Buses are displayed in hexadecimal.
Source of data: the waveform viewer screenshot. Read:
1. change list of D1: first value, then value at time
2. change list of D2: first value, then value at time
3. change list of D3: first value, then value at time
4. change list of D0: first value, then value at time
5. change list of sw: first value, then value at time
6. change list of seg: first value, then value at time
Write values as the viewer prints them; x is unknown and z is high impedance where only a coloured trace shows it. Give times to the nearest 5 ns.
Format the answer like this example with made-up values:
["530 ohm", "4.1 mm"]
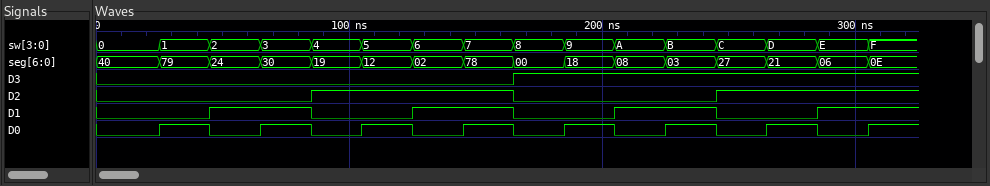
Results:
["0, 1 at 45 ns, 0 at 85 ns, 1 at 125 ns, 0 at 165 ns, 1 at 205 ns, 0 at 245 ns, 1 at 285 ns", "0, 1 at 85 ns, 0 at 165 ns, 1 at 245 ns", "0, 1 at 165 ns", "0, 1 at 25 ns, 0 at 45 ns, 1 at 65 ns, 0 at 85 ns, 1 at 105 ns, 0 at 125 ns, 1 at 145 ns, 0 at 165 ns, 1 at 185 ns, 0 at 205 ns, 1 at 225 ns, 0 at 245 ns, 1 at 265 ns, 0 at 285 ns, 1 at 305 ns", "0, 1 at 25 ns, 2 at 45 ns, 3 at 65 ns, 4 at 85 ns, 5 at 105 ns, 6 at 125 ns, 7 at 145 ns, 8 at 165 ns, 9 at 185 ns, A at 205 ns, B at 225 ns, C at 245 ns, D at 265 ns, E at 285 ns, F at 305 ns", "40, 79 at 25 ns, 24 at 45 ns, 30 at 65 ns, 19 at 85 ns, 12 at 105 ns, 02 at 125 ns, 78 at 145 ns, 00 at 165 ns, 18 at 185 ns, 08 at 205 ns, 03 at 225 ns, 27 at 245 ns, 21 at 265 ns, 06 at 285 ns, 0E at 305 ns"]
